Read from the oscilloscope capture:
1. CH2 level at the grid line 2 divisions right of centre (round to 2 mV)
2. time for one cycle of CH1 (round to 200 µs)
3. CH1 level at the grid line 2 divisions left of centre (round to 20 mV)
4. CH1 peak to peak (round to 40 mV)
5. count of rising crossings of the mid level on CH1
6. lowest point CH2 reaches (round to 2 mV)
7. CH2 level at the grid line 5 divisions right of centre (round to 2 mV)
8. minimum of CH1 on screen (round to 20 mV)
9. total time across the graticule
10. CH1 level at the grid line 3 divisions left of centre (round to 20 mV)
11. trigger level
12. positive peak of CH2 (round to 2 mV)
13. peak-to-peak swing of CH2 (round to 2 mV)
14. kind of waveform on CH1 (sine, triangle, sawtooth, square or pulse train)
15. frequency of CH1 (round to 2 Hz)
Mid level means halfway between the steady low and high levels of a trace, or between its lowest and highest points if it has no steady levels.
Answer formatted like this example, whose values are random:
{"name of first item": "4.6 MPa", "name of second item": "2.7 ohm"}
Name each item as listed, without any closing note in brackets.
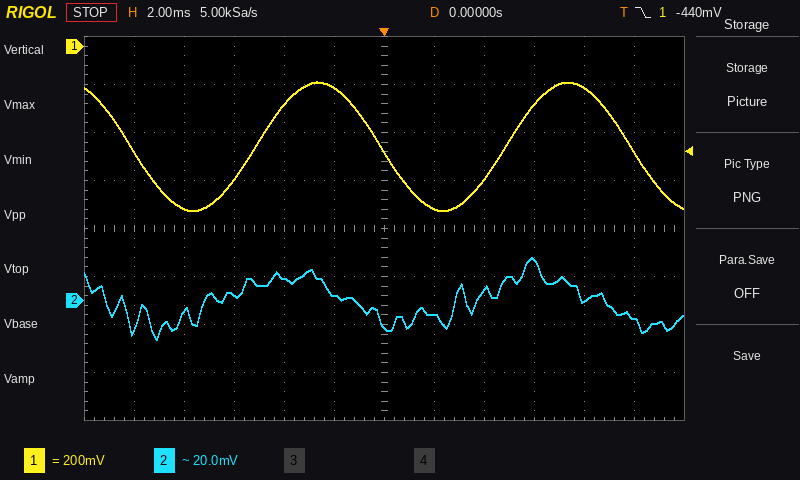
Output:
{"CH2 level at the grid line 2 divisions right of centre": "4 mV", "time for one cycle of CH1": "10.0 ms", "CH1 level at the grid line 2 divisions left of centre": "-240 mV", "CH1 peak to peak": "520 mV", "count of rising crossings of the mid level on CH1": "2", "lowest point CH2 reaches": "-16 mV", "CH2 level at the grid line 5 divisions right of centre": "-8 mV", "minimum of CH1 on screen": "-680 mV", "total time across the graticule": "24 ms", "CH1 level at the grid line 3 divisions left of centre": "-560 mV", "trigger level": "-440 mV", "positive peak of CH2": "18 mV", "peak-to-peak swing of CH2": "34 mV", "kind of waveform on CH1": "sine", "frequency of CH1": "100 Hz"}
